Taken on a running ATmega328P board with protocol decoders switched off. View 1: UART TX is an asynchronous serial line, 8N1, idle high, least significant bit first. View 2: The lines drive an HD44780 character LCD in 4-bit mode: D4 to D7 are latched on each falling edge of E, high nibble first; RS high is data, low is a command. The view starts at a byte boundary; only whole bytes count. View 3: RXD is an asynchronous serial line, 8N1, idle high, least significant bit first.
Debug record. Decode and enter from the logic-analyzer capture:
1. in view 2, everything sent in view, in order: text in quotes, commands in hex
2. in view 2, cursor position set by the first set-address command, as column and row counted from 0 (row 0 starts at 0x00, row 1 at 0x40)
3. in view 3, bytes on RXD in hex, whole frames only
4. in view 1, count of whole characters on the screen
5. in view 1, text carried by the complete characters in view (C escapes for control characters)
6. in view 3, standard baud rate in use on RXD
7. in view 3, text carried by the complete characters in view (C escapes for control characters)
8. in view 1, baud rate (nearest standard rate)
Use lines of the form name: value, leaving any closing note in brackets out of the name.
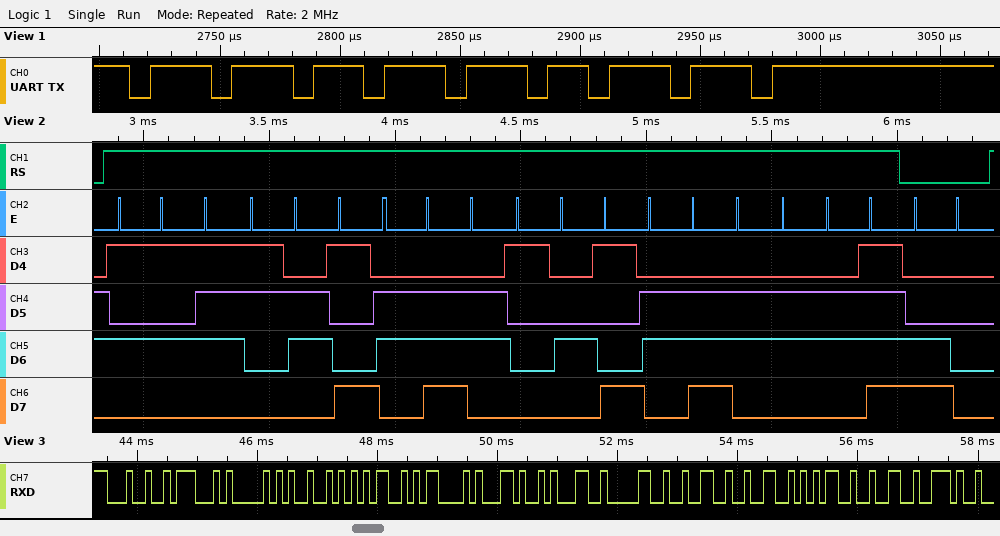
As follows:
in view 2, everything sent in view, in order: text in quotes, commands in hex: "UsinaInfo" 0xC0
in view 2, cursor position set by the first set-address command, as column and row counted from 0: column 0, row 1
in view 3, bytes on RXD in hex, whole frames only: 24 47 50 52 4D 43 2C 31 30 32 32 35 32 2E
in view 1, count of whole characters on the screen: 3
in view 1, text carried by the complete characters in view: "www"
in view 3, standard baud rate in use on RXD: 9600 baud
in view 3, text carried by the complete characters in view: "$GPRMC,102252."
in view 1, baud rate: 115200 baud
